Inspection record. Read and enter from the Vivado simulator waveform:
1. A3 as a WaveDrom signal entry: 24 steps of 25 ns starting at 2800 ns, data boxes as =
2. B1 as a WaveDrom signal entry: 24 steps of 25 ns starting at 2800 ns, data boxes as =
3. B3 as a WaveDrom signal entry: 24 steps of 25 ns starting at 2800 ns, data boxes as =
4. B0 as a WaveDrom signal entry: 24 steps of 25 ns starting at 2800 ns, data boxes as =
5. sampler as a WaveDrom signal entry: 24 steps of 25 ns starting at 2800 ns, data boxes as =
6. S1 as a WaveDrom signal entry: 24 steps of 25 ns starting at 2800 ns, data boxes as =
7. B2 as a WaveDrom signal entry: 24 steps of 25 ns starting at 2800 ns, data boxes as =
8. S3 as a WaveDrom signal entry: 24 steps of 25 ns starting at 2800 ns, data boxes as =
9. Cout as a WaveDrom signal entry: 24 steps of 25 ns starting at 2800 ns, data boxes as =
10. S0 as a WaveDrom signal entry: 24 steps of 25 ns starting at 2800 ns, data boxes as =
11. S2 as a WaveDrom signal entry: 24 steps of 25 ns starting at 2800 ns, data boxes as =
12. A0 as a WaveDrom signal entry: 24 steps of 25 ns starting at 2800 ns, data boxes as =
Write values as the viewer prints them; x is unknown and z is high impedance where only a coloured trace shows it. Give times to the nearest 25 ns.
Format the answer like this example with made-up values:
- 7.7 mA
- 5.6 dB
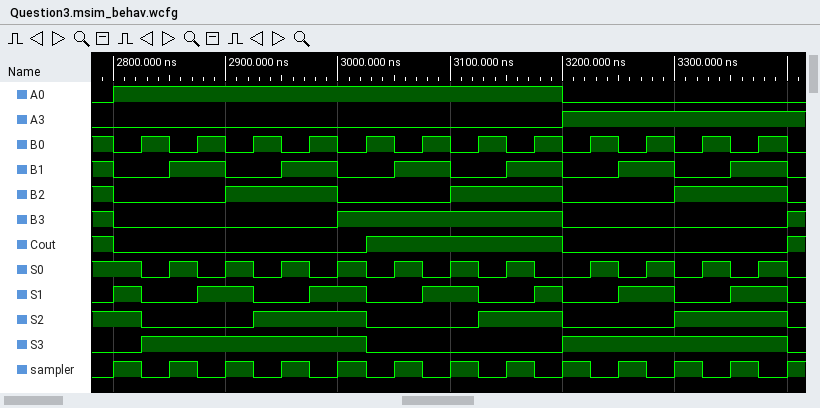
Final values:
- {name: 'A3', wave: '0...............1.......'}
- {name: 'B1', wave: '0.1.0.1.0.1.0.1.0.1.0.1.'}
- {name: 'B3', wave: '0.......1.......0.......'}
- {name: 'B0', wave: '010101010101010101010101'}
- {name: 'sampler', wave: '101010101010101010101010'}
- {name: 'S1', wave: '10.1.0.1.0.1.0.10.1.0.1.'}
- {name: 'B2', wave: '0...1...0...1...0...1...'}
- {name: 'S3', wave: '01.......0......1.......'}
- {name: 'Cout', wave: '0........1......0.......'}
- {name: 'S0', wave: '1010101010101010.1010101'}
- {name: 'S2', wave: '10...1...0...1..0...1...'}
- {name: 'A0', wave: '1...............0.......'}
